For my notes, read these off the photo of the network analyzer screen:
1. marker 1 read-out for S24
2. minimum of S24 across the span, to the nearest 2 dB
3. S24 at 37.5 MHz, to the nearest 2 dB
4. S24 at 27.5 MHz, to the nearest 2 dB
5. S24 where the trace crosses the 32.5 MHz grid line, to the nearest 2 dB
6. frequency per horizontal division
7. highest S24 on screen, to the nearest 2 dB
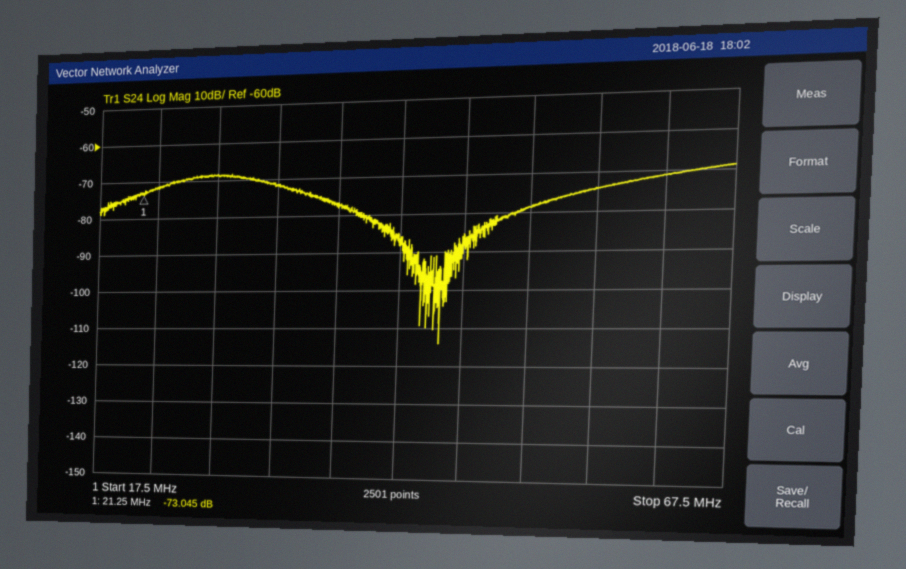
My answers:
-73.045 dB
-114 dB
-78 dB
-68 dB
-72 dB
5 MHz
-68 dB
